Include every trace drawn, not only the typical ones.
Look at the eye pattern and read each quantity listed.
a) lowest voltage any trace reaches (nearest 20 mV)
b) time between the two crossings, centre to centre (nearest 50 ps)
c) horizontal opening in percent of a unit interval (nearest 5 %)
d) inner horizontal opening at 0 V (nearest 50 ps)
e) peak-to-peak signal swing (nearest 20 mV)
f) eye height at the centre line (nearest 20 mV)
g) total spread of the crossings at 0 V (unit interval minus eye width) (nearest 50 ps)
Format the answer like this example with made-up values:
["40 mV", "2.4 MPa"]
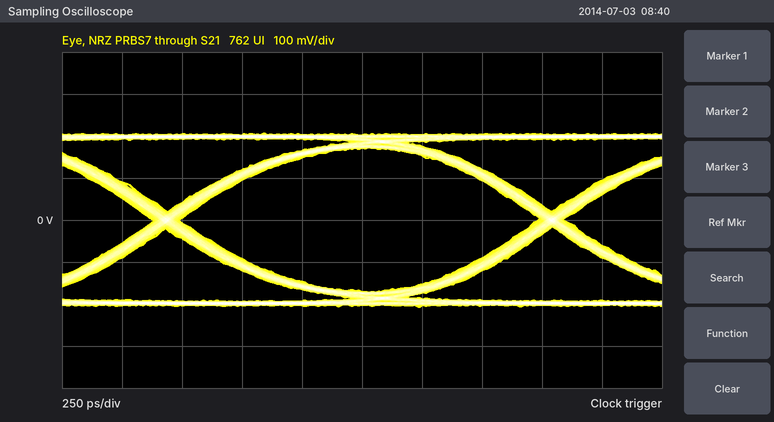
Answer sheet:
["-200 mV", "1.60 ns", "95 %", "1.50 ns", "420 mV", "340 mV", "100 ps"]
